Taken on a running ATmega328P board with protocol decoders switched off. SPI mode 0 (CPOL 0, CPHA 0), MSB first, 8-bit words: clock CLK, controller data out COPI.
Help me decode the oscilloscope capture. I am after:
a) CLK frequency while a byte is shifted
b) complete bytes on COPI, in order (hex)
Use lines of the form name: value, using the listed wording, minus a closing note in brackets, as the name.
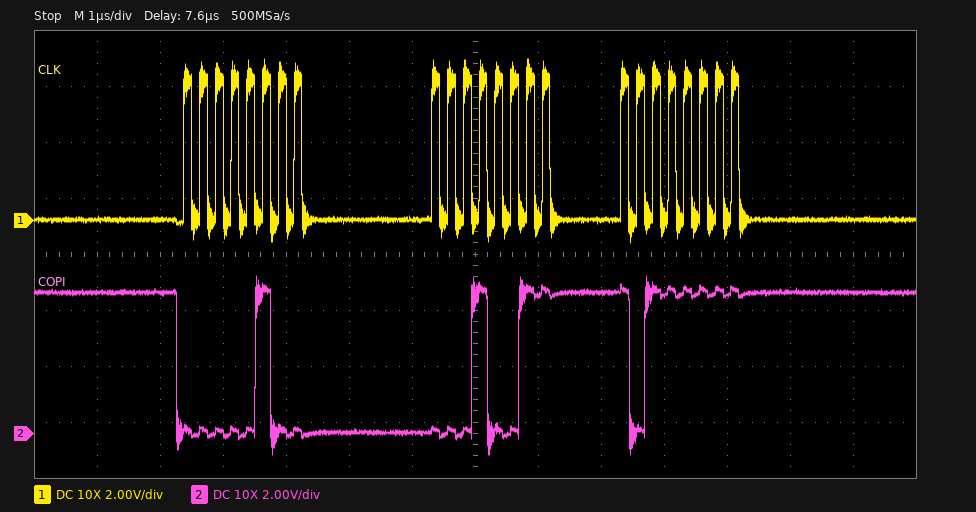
CLK frequency while a byte is shifted: 4 MHz
complete bytes on COPI, in order: 0x04 0x13 0xBF
